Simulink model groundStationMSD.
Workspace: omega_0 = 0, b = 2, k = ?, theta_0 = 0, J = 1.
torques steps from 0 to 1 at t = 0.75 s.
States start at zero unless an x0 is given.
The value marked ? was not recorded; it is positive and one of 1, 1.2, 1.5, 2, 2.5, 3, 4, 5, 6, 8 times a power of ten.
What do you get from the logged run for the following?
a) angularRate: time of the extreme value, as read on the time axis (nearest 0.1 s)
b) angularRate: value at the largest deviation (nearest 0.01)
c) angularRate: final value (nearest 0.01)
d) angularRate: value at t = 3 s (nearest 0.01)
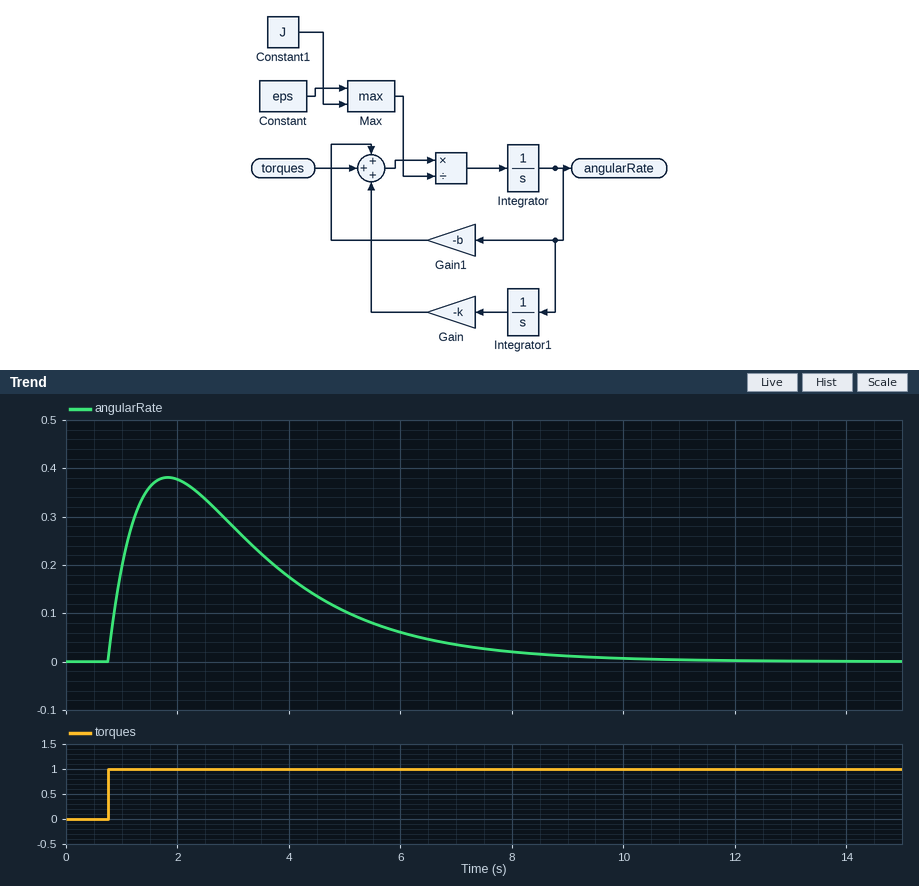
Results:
1.8 s
0.38
0.00
0.28
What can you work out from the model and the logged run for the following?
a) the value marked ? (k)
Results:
0.8
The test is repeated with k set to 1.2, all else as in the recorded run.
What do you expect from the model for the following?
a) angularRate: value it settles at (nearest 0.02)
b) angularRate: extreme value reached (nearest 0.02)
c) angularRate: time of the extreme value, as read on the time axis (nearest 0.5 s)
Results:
0.00
0.36
1.5 s
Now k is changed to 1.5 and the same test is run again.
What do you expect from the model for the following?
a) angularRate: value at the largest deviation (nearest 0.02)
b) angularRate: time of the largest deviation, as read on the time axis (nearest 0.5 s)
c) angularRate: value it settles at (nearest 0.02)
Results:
0.34
1.5 s
0.00
